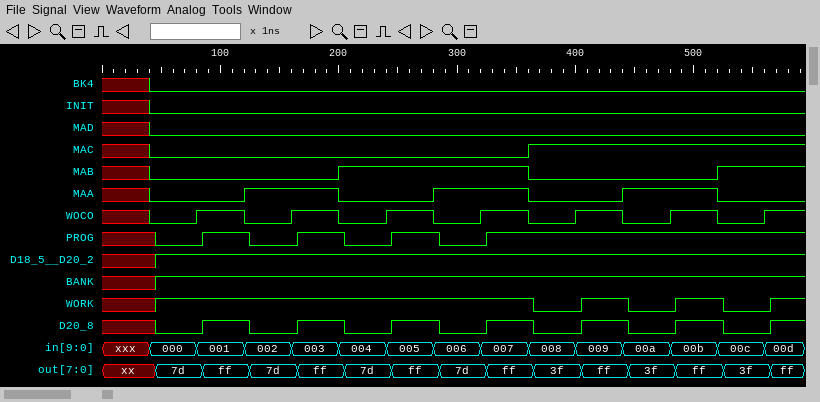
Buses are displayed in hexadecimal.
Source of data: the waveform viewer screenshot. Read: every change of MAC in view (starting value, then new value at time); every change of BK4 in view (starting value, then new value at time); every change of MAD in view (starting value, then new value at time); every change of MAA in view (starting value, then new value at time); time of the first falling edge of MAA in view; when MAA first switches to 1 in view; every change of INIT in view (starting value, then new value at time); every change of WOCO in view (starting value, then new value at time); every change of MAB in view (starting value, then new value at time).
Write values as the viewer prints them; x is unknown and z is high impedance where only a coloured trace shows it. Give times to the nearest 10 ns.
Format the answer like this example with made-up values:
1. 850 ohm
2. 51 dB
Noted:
1. x, 0 at 40 ns, 1 at 360 ns
2. x, 0 at 40 ns
3. x, 0 at 40 ns
4. x, 0 at 40 ns, 1 at 120 ns, 0 at 200 ns, 1 at 280 ns, 0 at 360 ns, 1 at 440 ns, 0 at 520 ns
5. 200 ns
6. 120 ns
7. x, 0 at 40 ns
8. x, 0 at 40 ns, 1 at 80 ns, 0 at 120 ns, 1 at 160 ns, 0 at 200 ns, 1 at 240 ns, 0 at 280 ns, 1 at 320 ns, 0 at 360 ns, 1 at 400 ns, 0 at 440 ns, 1 at 480 ns, 0 at 520 ns, 1 at 560 ns
9. x, 0 at 40 ns, 1 at 200 ns, 0 at 360 ns, 1 at 520 ns
